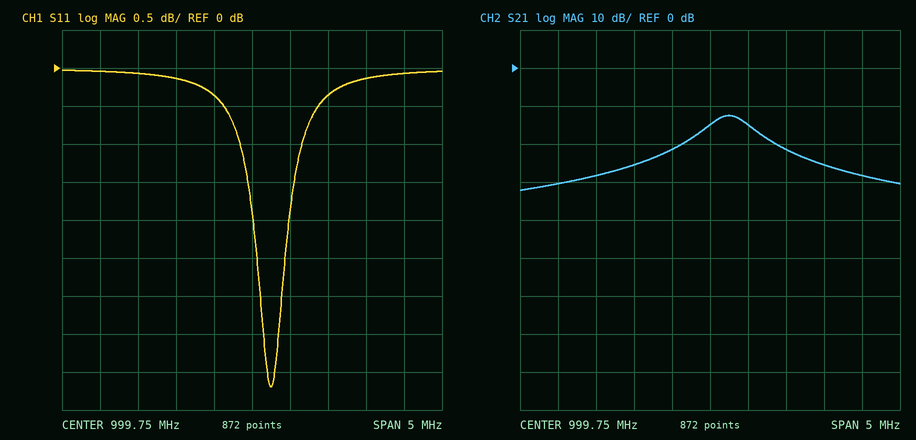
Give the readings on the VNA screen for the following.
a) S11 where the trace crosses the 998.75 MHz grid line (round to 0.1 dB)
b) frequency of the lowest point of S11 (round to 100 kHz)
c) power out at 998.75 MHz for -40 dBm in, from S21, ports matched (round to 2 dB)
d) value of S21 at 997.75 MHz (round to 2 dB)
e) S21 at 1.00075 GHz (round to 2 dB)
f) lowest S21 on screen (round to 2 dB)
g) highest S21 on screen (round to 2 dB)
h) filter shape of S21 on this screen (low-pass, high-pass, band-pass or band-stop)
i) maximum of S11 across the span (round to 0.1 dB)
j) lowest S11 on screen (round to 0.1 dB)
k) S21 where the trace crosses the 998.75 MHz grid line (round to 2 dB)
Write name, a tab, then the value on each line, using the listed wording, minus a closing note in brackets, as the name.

S11 where the trace crosses the 998.75 MHz grid line	-0.1 dB
frequency of the lowest point of S11	1.0000 GHz
power out at 998.75 MHz for -40 dBm in, from S21, ports matched	-66 dBm
value of S21 at 997.75 MHz	-30 dB
S21 at 1.00075 GHz	-22 dB
lowest S21 on screen	-32 dB
highest S21 on screen	-12 dB
filter shape of S21 on this screen	band-pass
maximum of S11 across the span	0.0 dB
lowest S11 on screen	-4.2 dB
S21 where the trace crosses the 998.75 MHz grid line	-26 dB
